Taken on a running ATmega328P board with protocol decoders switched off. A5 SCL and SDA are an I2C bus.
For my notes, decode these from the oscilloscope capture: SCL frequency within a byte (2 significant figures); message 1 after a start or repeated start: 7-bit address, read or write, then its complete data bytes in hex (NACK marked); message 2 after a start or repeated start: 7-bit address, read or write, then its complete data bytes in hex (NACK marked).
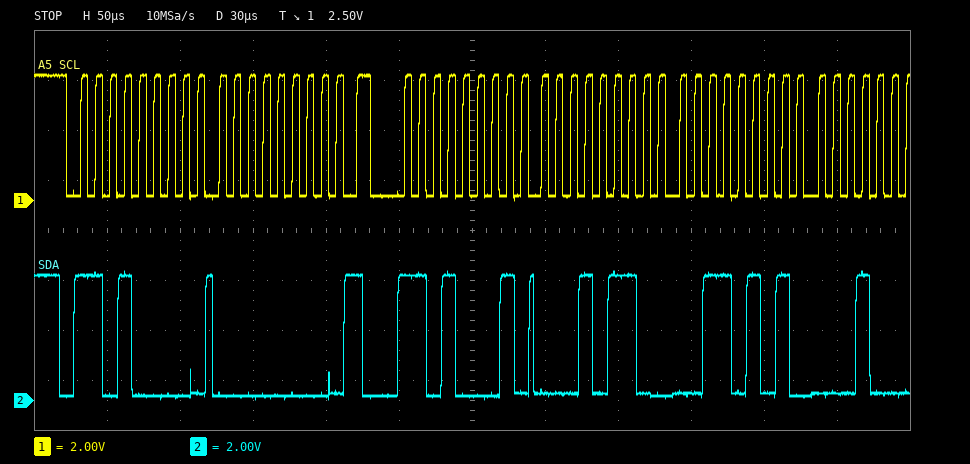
100 kHz
0x68 write: 00
0x68 read: 16 35
